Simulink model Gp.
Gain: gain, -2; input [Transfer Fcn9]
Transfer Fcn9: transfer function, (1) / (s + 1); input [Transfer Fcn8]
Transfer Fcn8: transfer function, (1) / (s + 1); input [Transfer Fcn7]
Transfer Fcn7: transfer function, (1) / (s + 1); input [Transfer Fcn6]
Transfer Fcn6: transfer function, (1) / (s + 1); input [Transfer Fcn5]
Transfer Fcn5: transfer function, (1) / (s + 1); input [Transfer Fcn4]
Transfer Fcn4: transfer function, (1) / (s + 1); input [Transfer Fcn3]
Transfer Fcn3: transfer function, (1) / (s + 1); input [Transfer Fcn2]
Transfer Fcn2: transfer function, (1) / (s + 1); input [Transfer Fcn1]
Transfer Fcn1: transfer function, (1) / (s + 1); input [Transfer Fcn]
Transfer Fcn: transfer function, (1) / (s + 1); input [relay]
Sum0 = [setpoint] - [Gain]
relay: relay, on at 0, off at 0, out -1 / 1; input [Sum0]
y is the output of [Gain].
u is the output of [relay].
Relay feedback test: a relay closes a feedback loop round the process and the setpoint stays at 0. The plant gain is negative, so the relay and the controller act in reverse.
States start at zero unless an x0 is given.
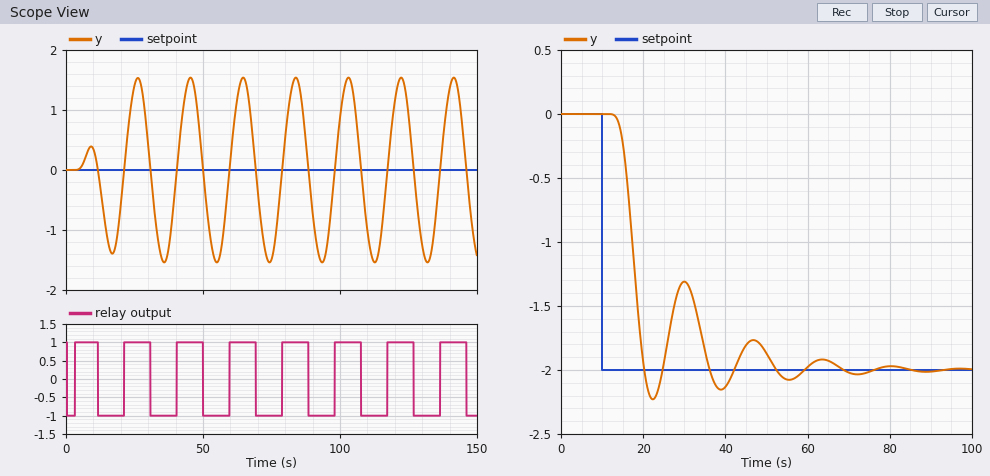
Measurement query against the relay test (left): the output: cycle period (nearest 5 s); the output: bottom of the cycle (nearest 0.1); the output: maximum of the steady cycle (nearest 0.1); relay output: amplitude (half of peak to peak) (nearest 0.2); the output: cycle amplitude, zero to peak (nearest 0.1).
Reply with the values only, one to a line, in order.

20 s
-1.5
1.5
1.0
1.5
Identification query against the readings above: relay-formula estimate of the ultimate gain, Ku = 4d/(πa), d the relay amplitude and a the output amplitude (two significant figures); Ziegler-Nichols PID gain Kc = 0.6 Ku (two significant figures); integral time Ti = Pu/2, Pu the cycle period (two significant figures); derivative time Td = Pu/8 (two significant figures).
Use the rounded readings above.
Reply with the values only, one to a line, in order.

0.85
0.51
10 s
2.5 s
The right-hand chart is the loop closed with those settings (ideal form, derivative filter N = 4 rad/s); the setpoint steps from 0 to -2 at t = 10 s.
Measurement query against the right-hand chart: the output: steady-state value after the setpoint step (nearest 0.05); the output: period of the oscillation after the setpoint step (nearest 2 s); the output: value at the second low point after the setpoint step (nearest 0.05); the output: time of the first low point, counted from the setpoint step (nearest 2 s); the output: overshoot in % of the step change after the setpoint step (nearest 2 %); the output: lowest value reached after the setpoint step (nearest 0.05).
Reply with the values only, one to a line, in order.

-2.00
16 s
-2.15
12 s
12 %
-2.25
